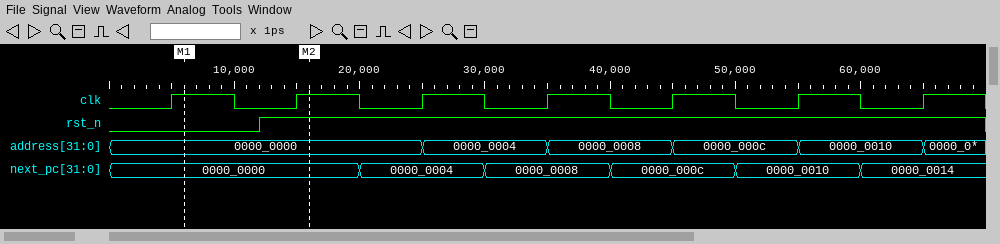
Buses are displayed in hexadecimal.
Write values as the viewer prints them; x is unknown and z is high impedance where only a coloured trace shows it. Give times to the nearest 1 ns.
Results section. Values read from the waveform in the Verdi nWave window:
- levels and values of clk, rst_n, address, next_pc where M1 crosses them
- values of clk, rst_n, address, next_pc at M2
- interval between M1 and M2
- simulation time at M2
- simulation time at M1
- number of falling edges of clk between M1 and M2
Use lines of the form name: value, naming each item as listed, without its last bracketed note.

levels and values of clk, rst_n, address, next_pc where M1 crosses them: clk=1, rst_n=0, address=0000_0000, next_pc=0000_0000
values of clk, rst_n, address, next_pc at M2: clk=1, rst_n=1, address=0000_0000, next_pc=0000_0000
interval between M1 and M2: 10 ns
simulation time at M2: 16 ns
simulation time at M1: 6 ns
number of falling edges of clk between M1 and M2: 1
